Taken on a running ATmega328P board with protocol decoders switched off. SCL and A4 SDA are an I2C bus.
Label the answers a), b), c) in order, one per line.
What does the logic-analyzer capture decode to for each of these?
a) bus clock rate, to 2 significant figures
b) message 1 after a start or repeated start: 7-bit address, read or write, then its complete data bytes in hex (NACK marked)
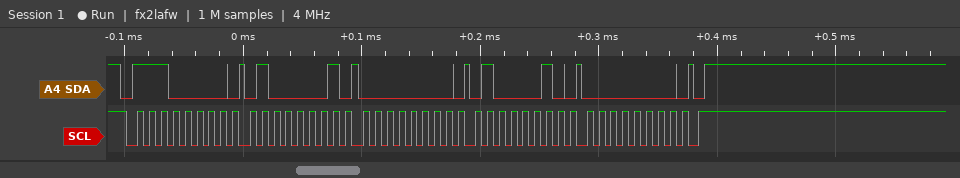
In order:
a) 100 kHz
b) 0x70 write: 41 00 42 00
